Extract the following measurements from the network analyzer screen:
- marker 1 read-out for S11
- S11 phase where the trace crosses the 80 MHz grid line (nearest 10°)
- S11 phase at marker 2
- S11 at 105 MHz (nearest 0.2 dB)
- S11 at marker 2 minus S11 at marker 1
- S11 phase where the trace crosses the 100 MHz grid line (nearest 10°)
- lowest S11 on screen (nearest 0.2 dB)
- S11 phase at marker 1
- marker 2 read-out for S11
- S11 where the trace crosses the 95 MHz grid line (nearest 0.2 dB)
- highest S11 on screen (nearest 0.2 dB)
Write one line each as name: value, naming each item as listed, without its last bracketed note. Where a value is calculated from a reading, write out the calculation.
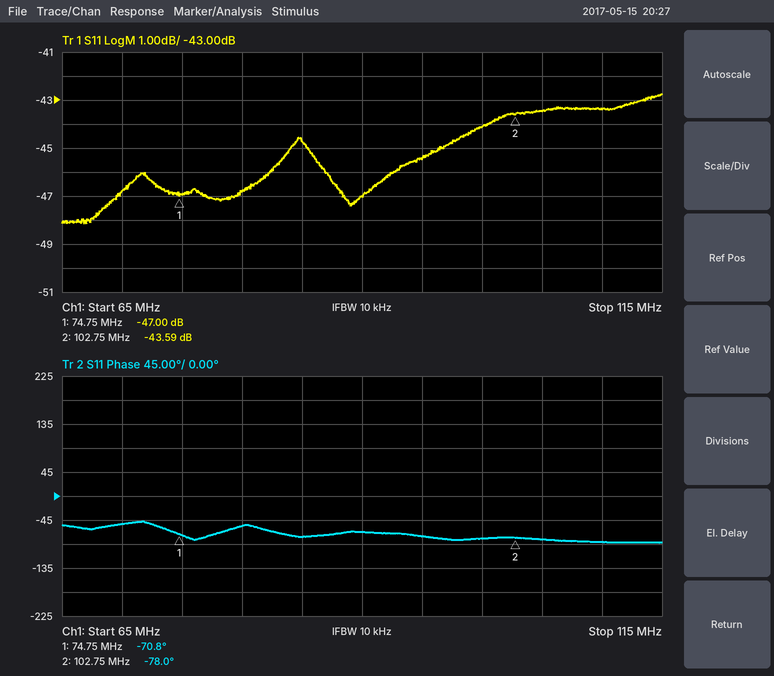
marker 1 read-out for S11: -47.00 dB
S11 phase where the trace crosses the 80 MHz grid line: -60°
S11 phase at marker 2: -78.0°
S11 at 105 MHz: -43.4 dB
S11 at marker 2 minus S11 at marker 1: -43.59 − (-47) = 3.41 dB
S11 phase where the trace crosses the 100 MHz grid line: -80°
lowest S11 on screen: -48.2 dB
S11 phase at marker 1: -70.8°
marker 2 read-out for S11: -43.59 dB
S11 where the trace crosses the 95 MHz grid line: -45.4 dB
highest S11 on screen: -42.8 dB
